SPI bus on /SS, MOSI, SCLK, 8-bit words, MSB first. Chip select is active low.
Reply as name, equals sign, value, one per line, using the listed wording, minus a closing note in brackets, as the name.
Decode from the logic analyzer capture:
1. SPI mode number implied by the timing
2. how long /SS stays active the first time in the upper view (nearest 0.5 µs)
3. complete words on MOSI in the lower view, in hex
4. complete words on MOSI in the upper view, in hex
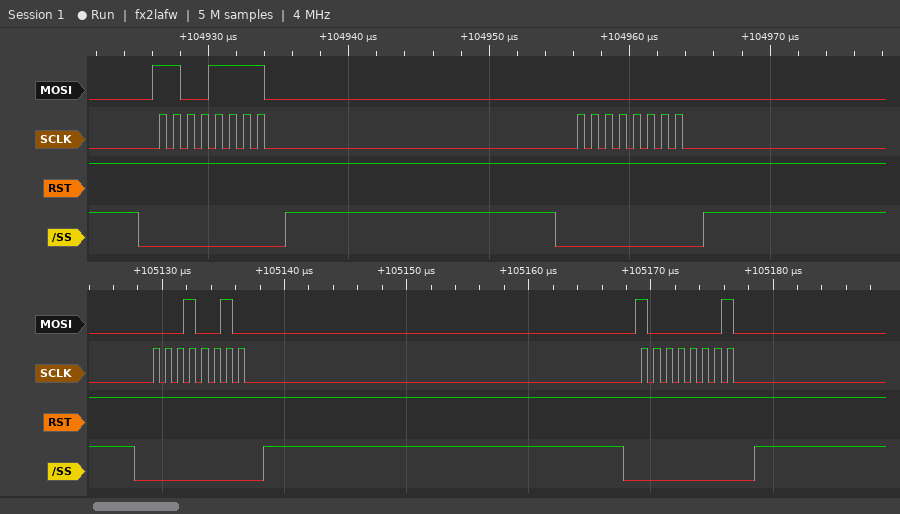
SPI mode number implied by the timing = 0
how long /SS stays active the first time in the upper view = 10.5 µs
complete words on MOSI in the lower view, in hex = 12, 81
complete words on MOSI in the upper view, in hex = CF, 00
